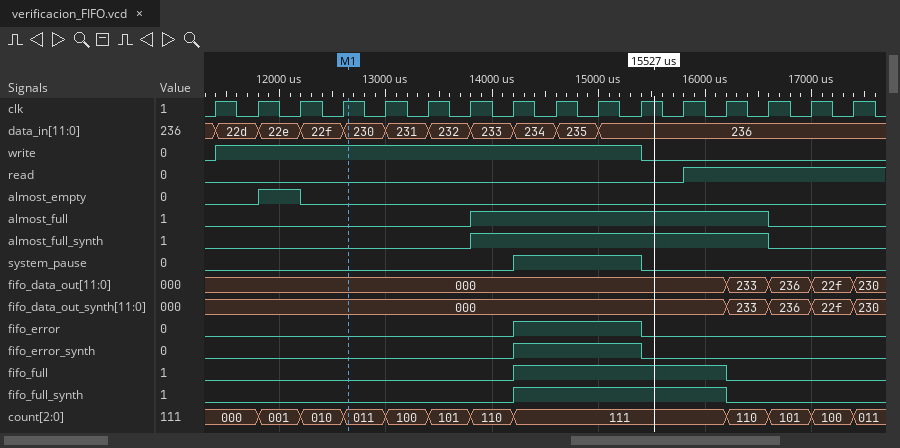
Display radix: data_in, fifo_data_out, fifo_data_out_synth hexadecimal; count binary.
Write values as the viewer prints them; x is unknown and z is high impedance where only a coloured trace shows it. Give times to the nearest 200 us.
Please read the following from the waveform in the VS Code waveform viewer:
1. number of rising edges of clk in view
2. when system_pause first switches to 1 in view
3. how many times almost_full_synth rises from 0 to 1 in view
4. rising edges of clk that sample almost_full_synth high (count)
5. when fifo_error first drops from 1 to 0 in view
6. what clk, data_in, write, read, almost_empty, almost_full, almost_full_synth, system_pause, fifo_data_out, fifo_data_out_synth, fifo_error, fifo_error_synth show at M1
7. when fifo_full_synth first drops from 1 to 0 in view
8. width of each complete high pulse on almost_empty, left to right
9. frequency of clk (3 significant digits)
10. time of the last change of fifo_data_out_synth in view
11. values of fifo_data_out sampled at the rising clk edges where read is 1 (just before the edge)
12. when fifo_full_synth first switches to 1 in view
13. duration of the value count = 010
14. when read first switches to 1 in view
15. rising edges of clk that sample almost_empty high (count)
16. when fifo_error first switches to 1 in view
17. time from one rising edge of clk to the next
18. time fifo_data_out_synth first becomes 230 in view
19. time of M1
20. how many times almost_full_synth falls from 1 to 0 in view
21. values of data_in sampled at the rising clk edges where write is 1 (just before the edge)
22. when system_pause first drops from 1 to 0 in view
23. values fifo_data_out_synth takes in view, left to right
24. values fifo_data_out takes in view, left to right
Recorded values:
16
14200 us
1
7
15400 us
clk=1, data_in=230, write=1, read=0, almost_empty=0, almost_full=0, almost_full_synth=0, system_pause=0, fifo_data_out=000, fifo_data_out_synth=000, fifo_error=0, fifo_error_synth=0
16200 us
400 us
2.50 kHz
17400 us
000, 233, 236, 22f
14200 us
400 us
15800 us
1
14200 us
400 us
17400 us
12600 us
1
22d, 22e, 22f, 230, 231, 232, 233, 234, 235, 236
15400 us
000, 233, 236, 22f, 230
000, 233, 236, 22f, 230
